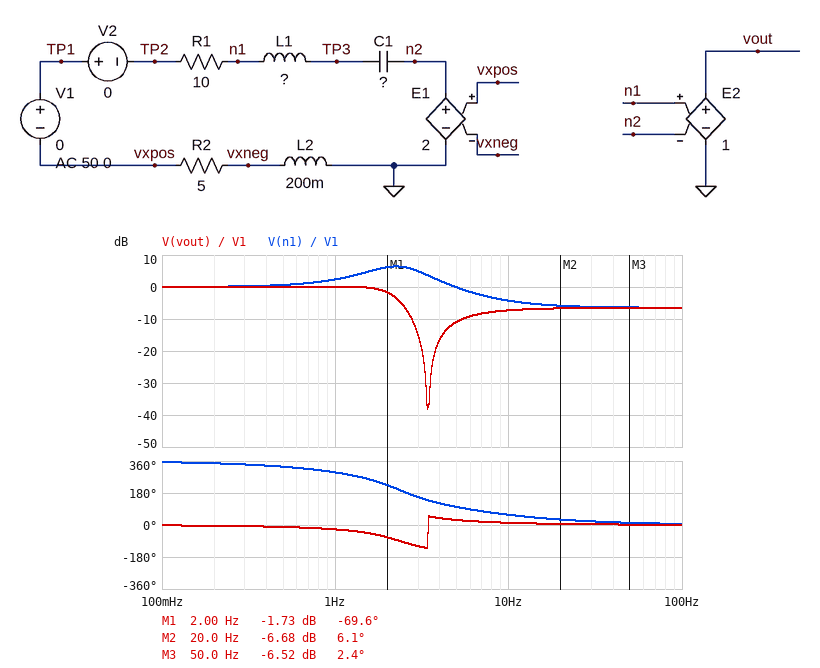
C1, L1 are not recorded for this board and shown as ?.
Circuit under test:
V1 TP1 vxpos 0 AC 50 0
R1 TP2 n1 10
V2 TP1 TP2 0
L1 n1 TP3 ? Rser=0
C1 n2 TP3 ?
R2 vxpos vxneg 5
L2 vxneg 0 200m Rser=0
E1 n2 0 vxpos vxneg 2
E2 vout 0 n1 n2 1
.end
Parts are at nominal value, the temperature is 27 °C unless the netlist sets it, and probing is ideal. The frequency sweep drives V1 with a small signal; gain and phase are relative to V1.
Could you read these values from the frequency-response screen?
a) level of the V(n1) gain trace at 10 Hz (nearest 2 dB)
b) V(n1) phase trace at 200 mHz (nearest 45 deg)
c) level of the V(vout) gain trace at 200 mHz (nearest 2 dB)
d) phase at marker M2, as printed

-4 dB
360 deg
0 dB
6.1 deg
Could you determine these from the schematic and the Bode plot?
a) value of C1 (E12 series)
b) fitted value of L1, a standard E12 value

12 mF
180 mH
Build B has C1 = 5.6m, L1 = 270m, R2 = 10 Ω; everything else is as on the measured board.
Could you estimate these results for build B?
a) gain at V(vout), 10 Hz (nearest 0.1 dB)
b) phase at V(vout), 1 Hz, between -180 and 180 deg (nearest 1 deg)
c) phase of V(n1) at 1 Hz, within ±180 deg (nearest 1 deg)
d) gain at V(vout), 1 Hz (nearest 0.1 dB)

-5.5 dB
0 deg
-37 deg
0.4 dB
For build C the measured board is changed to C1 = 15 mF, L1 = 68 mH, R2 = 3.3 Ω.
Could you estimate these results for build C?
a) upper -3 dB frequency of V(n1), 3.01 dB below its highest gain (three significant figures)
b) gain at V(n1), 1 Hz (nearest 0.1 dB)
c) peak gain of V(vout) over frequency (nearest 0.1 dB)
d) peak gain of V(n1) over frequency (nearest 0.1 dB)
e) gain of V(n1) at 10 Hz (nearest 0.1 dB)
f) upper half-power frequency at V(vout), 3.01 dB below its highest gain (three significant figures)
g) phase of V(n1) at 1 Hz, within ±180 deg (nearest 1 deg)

4.26 Hz
0.7 dB
0 dB
1.2 dB
-7.4 dB
1.79 Hz
-70 deg
